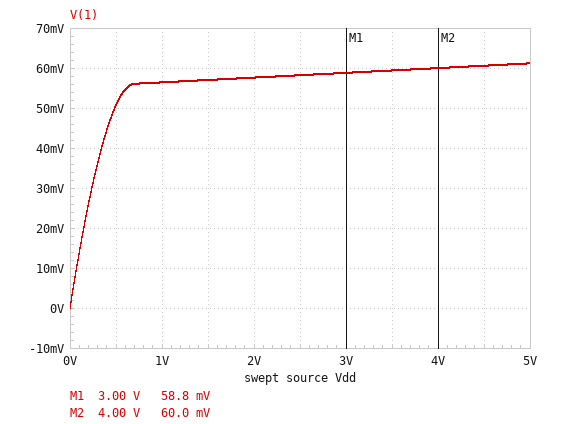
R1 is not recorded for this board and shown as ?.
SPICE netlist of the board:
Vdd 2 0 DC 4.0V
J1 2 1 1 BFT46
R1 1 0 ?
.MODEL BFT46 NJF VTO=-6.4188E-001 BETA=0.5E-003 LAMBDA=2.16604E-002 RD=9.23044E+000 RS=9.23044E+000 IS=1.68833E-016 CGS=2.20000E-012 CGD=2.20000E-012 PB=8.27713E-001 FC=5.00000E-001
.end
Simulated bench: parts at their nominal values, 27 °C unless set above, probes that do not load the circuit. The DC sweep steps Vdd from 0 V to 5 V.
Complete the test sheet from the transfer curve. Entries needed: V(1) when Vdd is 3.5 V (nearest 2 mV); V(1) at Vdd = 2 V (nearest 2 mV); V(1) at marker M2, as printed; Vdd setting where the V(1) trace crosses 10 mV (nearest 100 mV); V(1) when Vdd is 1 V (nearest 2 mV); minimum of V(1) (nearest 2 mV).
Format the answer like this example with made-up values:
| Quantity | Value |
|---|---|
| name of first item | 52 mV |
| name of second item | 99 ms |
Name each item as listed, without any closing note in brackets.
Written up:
| Quantity | Value |
|---|---|
| V(1) when Vdd is 3.5 V | 60 mV |
| V(1) at Vdd = 2 V | 58 mV |
| V(1) at marker M2, as printed | 60.0 mV |
| Vdd setting where the V(1) trace crosses 10 mV | 100 mV |
| V(1) when Vdd is 1 V | 56 mV |
| minimum of V(1) | 0 V |
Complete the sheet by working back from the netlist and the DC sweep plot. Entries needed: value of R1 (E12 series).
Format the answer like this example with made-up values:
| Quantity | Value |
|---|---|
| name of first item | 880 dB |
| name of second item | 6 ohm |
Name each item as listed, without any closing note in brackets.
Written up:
| Quantity | Value |
|---|---|
| value of R1 | 270 Ω |
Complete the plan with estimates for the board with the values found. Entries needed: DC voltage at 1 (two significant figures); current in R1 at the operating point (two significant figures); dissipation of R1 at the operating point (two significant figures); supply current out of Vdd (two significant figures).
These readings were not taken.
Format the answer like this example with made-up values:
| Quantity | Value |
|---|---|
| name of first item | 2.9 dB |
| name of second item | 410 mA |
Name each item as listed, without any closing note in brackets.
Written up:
| Quantity | Value |
|---|---|
| DC voltage at 1 | 60 mV |
| current in R1 at the operating point | 220 µA |
| dissipation of R1 at the operating point | 13 µW |
| supply current out of Vdd | 220 µA |
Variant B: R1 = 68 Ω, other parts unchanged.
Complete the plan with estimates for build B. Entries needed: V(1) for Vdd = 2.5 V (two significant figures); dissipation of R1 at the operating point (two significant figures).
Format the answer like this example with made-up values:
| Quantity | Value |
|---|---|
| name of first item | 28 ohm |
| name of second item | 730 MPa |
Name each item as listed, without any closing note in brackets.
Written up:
| Quantity | Value |
|---|---|
| V(1) for Vdd = 2.5 V | 15 mV |
| dissipation of R1 at the operating point | 3.4 µW |
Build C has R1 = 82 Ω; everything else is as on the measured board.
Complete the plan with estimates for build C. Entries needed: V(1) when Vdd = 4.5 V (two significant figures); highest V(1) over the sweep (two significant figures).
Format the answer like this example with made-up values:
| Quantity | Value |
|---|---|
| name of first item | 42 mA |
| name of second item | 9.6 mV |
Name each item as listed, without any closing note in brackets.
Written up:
| Quantity | Value |
|---|---|
| V(1) when Vdd = 4.5 V | 18 mV |
| highest V(1) over the sweep | 19 mV |
